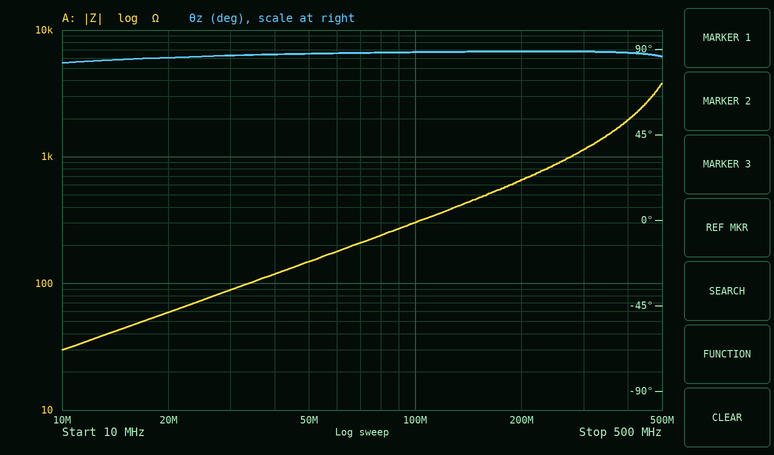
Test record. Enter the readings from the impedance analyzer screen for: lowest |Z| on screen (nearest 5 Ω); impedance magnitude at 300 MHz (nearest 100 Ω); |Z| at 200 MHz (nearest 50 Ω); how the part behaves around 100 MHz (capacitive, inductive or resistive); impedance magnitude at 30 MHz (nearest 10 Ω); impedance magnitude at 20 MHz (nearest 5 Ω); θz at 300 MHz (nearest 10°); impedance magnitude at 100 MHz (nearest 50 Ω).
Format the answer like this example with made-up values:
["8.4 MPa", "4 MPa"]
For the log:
["30 Ω", "1.1 kΩ", "650 Ω", "inductive", "90 Ω", "60 Ω", "90°", "300 Ω"]
